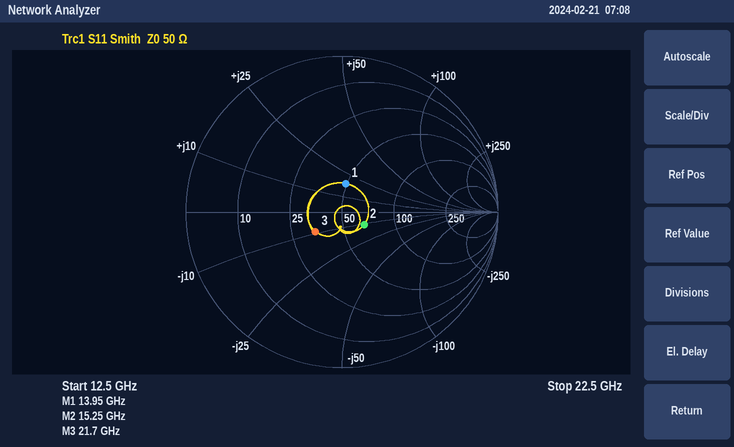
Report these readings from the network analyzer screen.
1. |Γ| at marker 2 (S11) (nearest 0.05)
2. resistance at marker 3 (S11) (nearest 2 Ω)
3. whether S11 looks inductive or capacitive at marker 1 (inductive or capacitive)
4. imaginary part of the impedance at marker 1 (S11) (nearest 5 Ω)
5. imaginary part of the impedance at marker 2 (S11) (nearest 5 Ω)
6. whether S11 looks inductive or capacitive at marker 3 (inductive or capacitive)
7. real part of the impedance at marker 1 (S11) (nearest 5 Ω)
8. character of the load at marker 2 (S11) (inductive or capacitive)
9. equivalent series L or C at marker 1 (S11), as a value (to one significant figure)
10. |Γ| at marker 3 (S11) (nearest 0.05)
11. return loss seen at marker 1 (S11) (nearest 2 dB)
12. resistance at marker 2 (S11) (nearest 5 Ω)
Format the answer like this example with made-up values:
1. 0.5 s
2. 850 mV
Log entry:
1. 0.15
2. 34 Ω
3. inductive
4. +20 Ω
5. -10 Ω
6. capacitive
7. 50 Ω
8. capacitive
9. 200 pH
10. 0.20
11. 14 dB
12. 65 Ω
